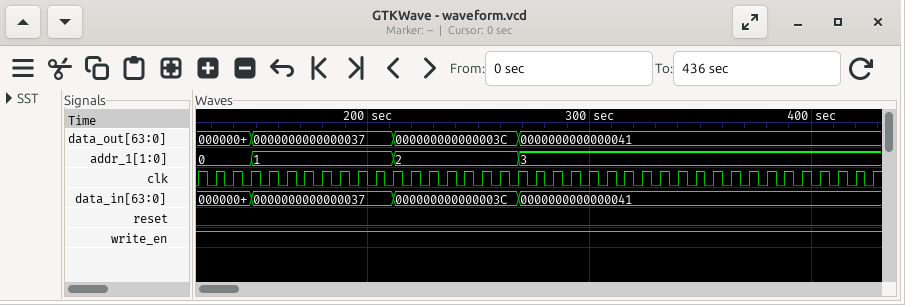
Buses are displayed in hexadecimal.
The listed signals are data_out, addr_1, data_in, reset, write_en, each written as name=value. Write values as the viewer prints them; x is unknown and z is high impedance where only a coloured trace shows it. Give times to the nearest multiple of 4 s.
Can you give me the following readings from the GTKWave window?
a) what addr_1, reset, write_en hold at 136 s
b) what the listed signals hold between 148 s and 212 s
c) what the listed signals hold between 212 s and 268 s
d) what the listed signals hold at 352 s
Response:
addr_1=0, reset=0, write_en=1
data_out=0000000000000037, addr_1=1, data_in=0000000000000037, reset=0, write_en=1
data_out=000000000000003C, addr_1=2, data_in=000000000000003C, reset=0, write_en=1
data_out=0000000000000041, addr_1=3, data_in=0000000000000041, reset=0, write_en=1
